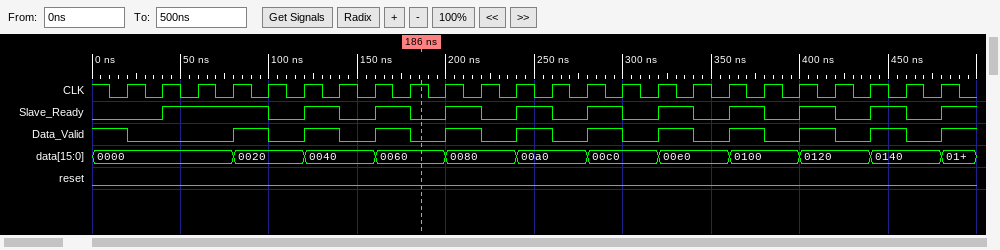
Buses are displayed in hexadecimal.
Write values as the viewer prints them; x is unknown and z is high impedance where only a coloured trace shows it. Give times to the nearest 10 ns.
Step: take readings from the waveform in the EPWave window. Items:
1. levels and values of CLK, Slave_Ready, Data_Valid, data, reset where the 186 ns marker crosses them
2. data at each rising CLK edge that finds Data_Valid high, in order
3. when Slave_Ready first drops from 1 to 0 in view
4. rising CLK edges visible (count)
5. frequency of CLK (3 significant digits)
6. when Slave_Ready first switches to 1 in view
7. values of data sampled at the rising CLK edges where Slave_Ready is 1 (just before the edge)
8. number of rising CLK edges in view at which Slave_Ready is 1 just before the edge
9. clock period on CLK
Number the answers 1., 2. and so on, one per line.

1. CLK=1, Slave_Ready=0, Data_Valid=0, data=0060, reset=0
2. 0000, 0020, 0040, 0060, 0080, 00a0, 00c0, 00e0, 0100, 0120, 0140
3. 100 ns
4. 24
5. 50.0 MHz
6. 40 ns
7. 0000, 0000, 0020, 0040, 0060, 0080, 00a0, 00c0, 00e0, 0100, 0120, 0140
8. 12
9. 20 ns
